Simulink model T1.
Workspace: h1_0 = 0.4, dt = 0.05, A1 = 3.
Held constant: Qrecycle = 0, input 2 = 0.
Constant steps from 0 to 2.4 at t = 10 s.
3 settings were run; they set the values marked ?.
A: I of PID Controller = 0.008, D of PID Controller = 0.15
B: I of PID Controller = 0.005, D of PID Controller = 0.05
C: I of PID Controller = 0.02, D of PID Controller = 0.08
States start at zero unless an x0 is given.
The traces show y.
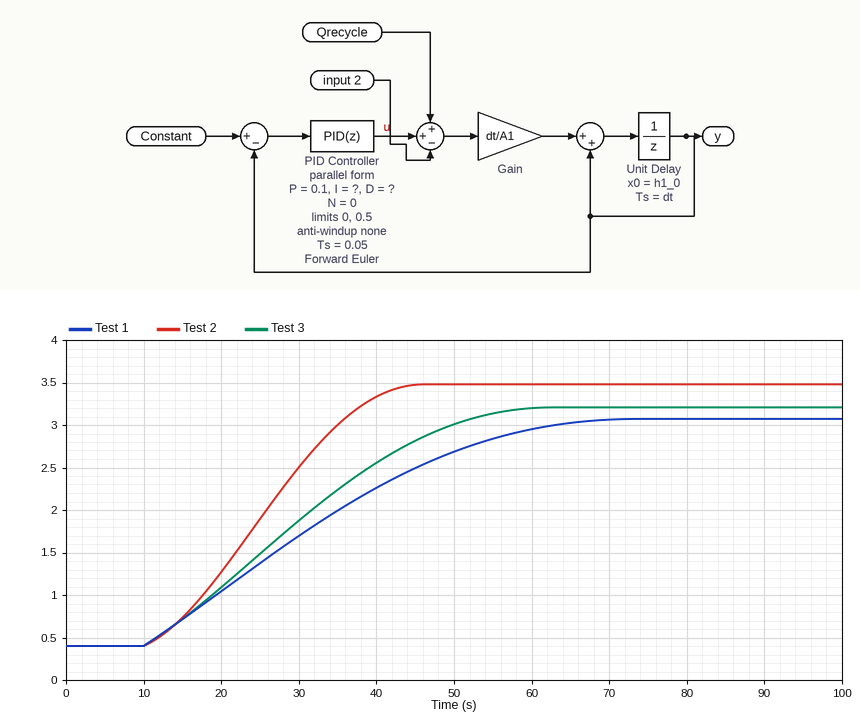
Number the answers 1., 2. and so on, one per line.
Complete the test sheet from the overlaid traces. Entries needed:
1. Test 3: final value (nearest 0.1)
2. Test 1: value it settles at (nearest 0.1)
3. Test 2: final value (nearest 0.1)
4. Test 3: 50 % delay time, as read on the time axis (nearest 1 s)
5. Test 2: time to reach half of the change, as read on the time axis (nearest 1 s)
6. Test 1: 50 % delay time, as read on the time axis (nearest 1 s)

1. 3.2
2. 3.1
3. 3.5
4. 29 s
5. 25 s
6. 31 s
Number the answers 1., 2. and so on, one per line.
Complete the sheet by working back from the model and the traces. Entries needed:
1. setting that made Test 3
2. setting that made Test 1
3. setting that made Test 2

1. A
2. B
3. C
